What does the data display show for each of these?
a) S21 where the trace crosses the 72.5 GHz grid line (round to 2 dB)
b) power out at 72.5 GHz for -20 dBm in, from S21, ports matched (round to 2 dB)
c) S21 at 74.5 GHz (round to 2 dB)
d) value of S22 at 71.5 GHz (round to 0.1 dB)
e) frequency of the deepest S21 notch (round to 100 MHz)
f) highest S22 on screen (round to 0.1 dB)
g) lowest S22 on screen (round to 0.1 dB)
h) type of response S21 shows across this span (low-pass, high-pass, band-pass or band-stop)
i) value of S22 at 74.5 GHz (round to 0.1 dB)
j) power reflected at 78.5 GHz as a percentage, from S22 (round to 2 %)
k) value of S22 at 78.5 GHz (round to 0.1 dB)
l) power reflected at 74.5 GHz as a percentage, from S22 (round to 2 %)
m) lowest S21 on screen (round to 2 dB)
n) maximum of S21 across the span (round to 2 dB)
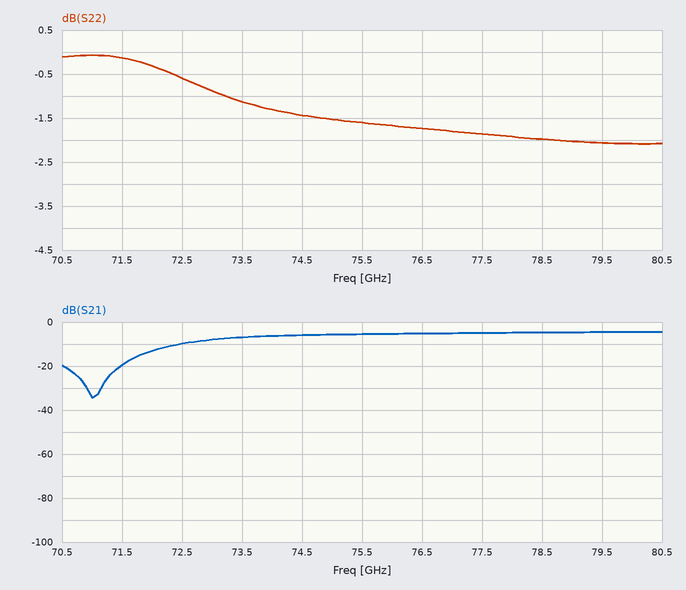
-10 dB
-30 dBm
-6 dB
-0.1 dB
71.0 GHz
-0.1 dB
-2.1 dB
high-pass
-1.4 dB
64 %
-2.0 dB
72 %
-34 dB
-4 dB
